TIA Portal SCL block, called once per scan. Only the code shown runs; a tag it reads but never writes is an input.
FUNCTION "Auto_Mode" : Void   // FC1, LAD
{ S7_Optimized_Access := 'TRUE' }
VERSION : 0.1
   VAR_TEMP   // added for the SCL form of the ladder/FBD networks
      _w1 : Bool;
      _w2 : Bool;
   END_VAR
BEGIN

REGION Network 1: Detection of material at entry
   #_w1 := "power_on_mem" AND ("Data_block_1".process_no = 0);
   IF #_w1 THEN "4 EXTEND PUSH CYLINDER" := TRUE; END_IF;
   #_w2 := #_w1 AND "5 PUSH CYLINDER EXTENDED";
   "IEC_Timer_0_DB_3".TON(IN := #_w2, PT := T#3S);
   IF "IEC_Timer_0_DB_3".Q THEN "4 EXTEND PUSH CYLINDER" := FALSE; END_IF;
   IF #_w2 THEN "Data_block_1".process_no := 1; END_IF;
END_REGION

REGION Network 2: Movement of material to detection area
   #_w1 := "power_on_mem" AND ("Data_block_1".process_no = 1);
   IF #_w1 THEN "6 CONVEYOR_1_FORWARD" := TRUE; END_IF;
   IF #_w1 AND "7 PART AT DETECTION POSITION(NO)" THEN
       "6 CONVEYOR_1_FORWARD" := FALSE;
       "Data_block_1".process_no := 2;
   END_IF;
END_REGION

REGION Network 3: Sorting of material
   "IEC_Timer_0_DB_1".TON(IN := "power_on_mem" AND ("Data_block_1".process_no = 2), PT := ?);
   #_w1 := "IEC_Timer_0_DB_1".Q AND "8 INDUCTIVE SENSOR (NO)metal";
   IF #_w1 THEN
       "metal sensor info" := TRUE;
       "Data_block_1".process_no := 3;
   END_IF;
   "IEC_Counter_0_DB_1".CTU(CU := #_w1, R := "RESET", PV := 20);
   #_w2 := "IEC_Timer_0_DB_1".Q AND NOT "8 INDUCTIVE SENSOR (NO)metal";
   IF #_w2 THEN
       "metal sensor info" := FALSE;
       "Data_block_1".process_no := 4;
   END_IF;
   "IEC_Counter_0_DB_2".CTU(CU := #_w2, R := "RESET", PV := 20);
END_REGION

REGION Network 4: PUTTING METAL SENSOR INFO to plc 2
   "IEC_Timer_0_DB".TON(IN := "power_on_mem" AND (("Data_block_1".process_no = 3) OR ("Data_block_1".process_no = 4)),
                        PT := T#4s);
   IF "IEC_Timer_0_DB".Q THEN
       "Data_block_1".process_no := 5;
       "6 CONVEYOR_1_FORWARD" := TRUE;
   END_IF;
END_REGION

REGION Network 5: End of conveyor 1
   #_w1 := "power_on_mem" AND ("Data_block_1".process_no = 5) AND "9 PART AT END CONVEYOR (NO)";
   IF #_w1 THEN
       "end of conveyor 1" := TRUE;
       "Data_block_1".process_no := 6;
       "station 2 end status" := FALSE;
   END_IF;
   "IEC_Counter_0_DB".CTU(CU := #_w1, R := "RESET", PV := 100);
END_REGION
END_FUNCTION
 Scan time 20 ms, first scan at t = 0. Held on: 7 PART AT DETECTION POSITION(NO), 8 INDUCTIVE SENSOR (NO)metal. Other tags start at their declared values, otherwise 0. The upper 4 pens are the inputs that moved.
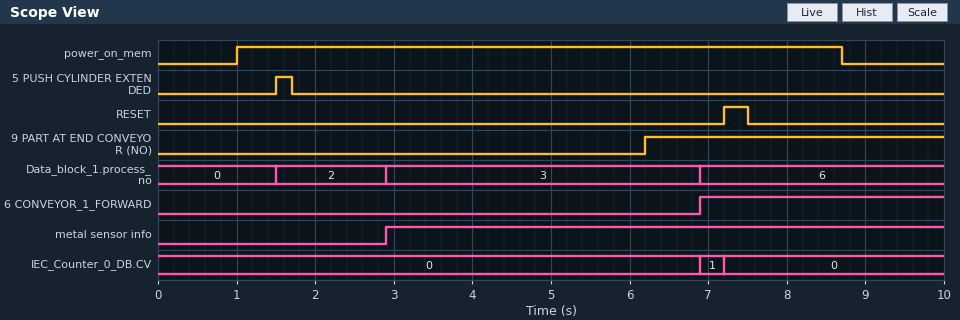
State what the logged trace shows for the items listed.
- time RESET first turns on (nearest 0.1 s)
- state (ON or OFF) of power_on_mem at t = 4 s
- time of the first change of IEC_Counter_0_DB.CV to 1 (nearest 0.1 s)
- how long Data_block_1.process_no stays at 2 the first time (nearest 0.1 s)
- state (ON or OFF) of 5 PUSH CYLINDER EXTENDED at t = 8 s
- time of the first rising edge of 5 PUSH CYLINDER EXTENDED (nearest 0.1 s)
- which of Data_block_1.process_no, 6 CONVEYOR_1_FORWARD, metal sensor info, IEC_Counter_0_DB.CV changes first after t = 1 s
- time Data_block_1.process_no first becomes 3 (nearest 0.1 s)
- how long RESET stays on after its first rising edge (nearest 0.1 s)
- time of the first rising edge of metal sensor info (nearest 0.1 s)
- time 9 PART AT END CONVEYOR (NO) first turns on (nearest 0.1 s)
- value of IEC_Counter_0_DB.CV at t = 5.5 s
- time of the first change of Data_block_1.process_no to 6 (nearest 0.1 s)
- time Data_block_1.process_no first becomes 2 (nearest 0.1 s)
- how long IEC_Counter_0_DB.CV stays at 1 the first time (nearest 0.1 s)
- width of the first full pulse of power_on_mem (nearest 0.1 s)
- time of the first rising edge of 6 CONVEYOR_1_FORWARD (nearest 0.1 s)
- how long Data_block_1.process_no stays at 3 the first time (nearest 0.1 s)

7.2 s
ON
6.9 s
1.4 s
OFF
1.5 s
Data_block_1.process_no
2.9 s
0.3 s
2.9 s
6.2 s
0
6.9 s
1.5 s
0.3 s
7.7 s
6.9 s
4.0 s
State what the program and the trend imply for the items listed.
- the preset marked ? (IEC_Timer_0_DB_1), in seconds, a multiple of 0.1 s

1.4 s
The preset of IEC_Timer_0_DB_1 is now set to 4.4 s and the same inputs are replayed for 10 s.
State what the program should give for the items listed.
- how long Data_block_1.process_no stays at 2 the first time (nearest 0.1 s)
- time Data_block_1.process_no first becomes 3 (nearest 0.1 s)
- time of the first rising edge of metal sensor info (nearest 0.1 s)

4.4 s
5.9 s
5.9 s
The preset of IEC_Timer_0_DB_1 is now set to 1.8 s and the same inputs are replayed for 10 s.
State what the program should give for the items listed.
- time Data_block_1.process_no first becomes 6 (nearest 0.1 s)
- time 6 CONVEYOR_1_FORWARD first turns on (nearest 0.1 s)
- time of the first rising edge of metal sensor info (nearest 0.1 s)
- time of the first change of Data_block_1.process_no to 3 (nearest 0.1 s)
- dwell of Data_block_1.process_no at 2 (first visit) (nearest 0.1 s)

7.3 s
7.3 s
3.3 s
3.3 s
1.8 s
